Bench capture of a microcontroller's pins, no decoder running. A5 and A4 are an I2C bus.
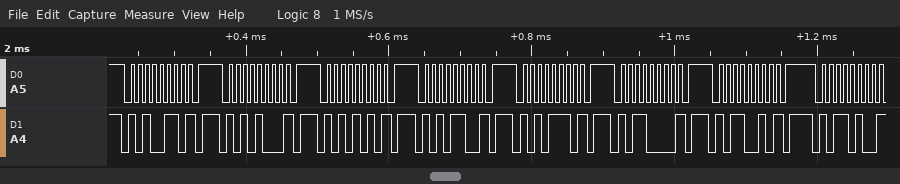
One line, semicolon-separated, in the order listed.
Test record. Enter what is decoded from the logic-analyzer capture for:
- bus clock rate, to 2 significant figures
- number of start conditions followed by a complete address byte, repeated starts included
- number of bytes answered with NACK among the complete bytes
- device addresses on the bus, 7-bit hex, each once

100 kHz; 8; 8; 0x53 0x54 0x55 0x56 0x57 0x58 0x59 0x5A
